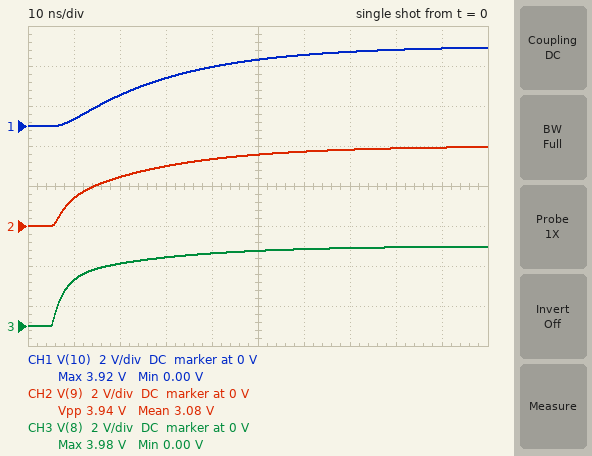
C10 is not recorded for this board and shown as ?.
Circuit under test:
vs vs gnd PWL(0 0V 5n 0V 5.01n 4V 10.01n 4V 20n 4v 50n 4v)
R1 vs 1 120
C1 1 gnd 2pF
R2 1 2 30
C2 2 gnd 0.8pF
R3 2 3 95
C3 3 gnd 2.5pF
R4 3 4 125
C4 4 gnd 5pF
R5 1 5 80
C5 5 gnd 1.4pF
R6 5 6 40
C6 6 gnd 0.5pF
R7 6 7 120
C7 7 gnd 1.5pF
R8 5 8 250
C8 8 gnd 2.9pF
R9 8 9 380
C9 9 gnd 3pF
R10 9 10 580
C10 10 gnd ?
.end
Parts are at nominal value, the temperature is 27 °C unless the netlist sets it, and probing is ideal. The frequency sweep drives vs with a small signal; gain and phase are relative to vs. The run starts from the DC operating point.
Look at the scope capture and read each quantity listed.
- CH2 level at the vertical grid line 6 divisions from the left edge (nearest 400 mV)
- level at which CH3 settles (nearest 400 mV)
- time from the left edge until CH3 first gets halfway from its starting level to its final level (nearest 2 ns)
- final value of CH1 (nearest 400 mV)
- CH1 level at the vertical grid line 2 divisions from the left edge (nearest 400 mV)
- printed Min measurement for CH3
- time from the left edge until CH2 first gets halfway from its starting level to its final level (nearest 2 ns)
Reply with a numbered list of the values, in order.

1. 3.6 V
2. 4.0 V
3. 8 ns
4. 4.0 V
5. 1.6 V
6. 0.00 V
7. 14 ns
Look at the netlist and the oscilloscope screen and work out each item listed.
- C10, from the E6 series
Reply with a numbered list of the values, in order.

1. 15 pF
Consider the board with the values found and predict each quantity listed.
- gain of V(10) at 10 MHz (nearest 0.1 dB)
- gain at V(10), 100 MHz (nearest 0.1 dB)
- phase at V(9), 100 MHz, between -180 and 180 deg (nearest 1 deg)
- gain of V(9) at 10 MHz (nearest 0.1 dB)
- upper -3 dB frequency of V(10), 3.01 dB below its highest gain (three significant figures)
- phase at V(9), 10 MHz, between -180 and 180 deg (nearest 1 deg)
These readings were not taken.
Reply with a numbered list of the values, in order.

1. -5.1 dB
2. -29.6 dB
3. -93 deg
4. -4.0 dB
5. 6.71 MHz
6. -39 deg
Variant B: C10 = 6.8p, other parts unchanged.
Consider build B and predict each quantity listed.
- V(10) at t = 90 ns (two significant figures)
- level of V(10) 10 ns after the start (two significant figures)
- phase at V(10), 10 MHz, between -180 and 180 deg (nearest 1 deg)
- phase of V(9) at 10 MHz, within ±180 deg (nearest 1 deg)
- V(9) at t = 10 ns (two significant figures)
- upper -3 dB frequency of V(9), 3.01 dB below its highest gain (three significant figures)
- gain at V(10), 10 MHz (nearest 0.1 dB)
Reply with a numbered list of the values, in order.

1. 4.0 V
2. 650 mV
3. -49 deg
4. -35 deg
5. 1.5 V
6. 14.0 MHz
7. -2.1 dB
